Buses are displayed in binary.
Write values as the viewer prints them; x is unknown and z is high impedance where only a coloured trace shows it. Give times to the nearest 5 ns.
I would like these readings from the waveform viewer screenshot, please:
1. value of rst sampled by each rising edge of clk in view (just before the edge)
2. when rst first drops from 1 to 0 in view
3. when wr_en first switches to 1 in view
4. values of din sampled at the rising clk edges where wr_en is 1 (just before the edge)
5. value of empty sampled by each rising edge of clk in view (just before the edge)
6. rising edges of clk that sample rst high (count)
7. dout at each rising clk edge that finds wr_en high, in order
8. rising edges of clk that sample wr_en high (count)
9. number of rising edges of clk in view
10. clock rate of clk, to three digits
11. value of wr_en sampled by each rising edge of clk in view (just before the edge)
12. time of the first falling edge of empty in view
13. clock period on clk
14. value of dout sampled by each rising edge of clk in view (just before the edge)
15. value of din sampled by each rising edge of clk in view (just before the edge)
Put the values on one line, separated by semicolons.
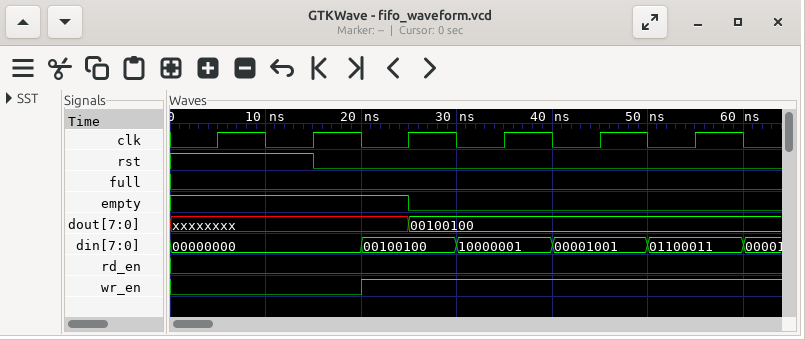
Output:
1 1 0 0 0 0; 15 ns; 20 ns; 00100100, 10000001, 00001001, 01100011; 1 1 1 0 0 0; 2; xxxxxxxx, 00100100, 00100100, 00100100; 4; 6; 100 MHz; 0 0 1 1 1 1; 25 ns; 10 ns; xxxxxxxx, xxxxxxxx, xxxxxxxx, 00100100, 00100100, 00100100; 00000000, 00000000, 00100100, 10000001, 00001001, 01100011
